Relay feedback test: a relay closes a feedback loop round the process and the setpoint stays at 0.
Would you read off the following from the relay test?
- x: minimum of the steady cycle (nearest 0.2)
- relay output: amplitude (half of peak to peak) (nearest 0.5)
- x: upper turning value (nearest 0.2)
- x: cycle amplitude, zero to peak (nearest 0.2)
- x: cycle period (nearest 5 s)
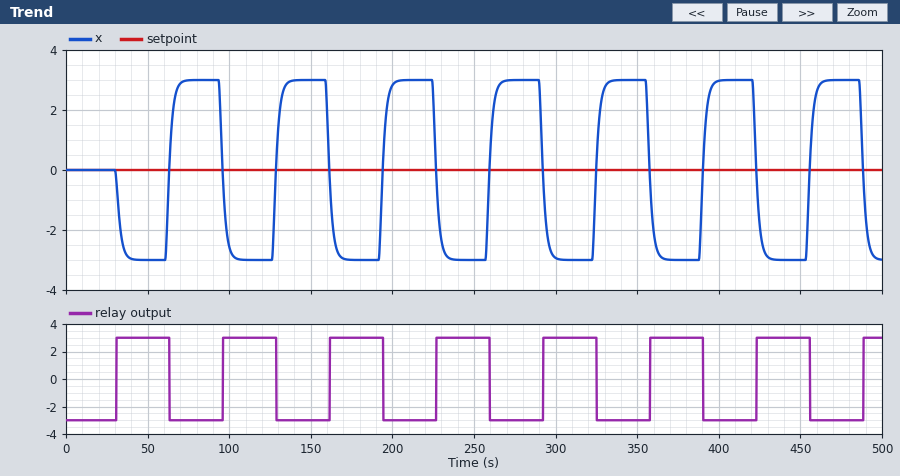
-3.0
3.0
3.0
3.0
65 s
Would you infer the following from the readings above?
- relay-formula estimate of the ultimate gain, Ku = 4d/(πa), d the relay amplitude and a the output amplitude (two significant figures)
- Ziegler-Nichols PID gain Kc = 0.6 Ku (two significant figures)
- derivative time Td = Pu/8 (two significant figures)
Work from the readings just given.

1.3
0.78
8.1 s
